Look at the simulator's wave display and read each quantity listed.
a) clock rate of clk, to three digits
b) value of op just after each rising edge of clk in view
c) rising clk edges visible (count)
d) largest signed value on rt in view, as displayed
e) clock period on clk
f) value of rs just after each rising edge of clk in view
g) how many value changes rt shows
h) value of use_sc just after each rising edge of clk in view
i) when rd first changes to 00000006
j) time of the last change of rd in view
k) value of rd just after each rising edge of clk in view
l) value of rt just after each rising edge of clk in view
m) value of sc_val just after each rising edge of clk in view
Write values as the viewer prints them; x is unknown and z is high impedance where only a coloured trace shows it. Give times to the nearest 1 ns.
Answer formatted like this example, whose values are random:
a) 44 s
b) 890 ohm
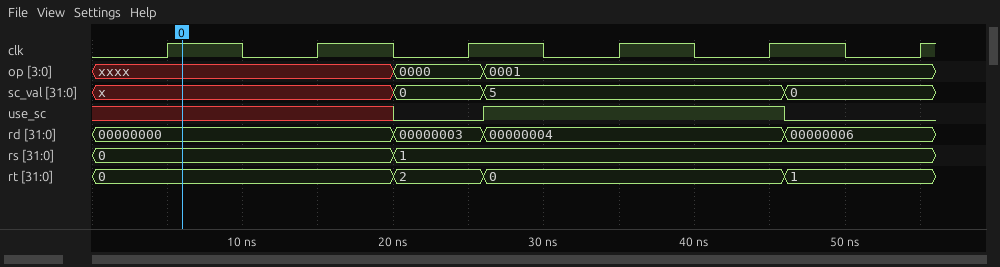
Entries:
a) 100 MHz
b) xxxx, xxxx, 0000, 0001, 0001, 0001
c) 6
d) 2
e) 10 ns
f) 0, 0, 1, 1, 1, 1
g) 3
h) x x 0 1 1 0
i) 46 ns
j) 46 ns
k) 00000000, 00000000, 00000003, 00000004, 00000004, 00000006
l) 0, 0, 2, 0, 0, 1
m) x, x, 0, 5, 5, 0
